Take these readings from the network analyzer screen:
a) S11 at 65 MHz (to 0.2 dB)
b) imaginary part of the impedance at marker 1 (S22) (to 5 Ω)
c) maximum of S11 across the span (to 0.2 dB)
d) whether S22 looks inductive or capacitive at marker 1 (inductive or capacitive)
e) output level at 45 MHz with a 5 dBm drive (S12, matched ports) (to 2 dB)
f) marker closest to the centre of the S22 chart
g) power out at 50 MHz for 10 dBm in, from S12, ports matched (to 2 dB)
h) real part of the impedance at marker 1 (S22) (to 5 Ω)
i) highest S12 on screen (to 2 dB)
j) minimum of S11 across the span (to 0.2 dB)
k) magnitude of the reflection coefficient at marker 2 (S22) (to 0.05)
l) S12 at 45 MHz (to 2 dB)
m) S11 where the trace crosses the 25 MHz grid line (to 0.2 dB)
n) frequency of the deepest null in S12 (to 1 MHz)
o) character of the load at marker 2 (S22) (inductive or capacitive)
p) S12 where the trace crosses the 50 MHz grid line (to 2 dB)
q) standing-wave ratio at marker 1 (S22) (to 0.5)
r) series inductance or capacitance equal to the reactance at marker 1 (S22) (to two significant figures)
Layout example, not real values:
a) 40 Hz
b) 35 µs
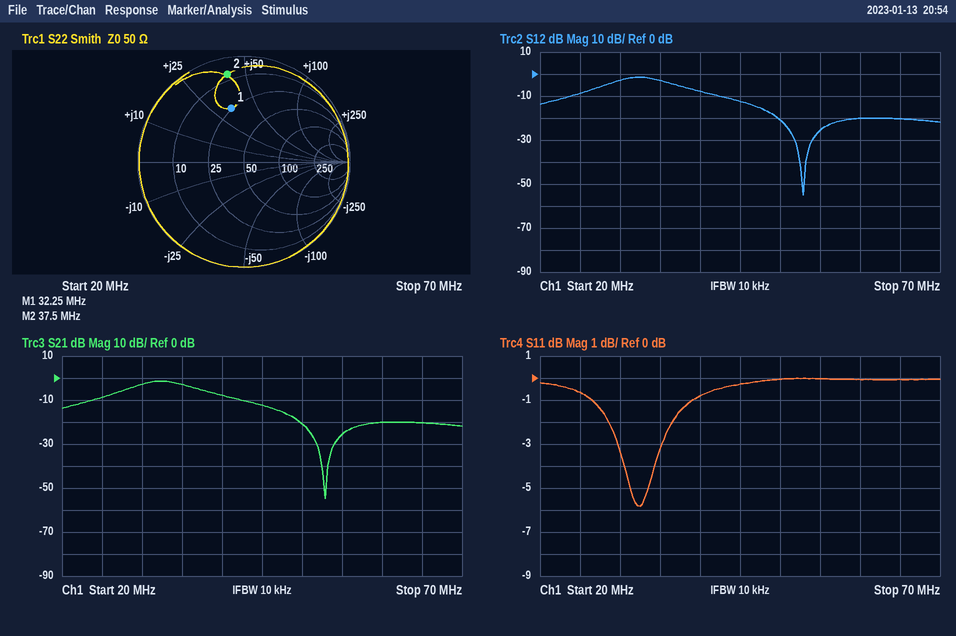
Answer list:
a) 0.0 dB
b) +35 Ω
c) 0.0 dB
d) inductive
e) -8 dBm
f) marker 1
g) -10 dBm
h) 25 Ω
i) -2 dB
j) -5.8 dB
k) 0.85
l) -12 dB
m) -0.6 dB
n) 53 MHz
o) inductive
p) -20 dB
q) 3.0
r) 170 nH
